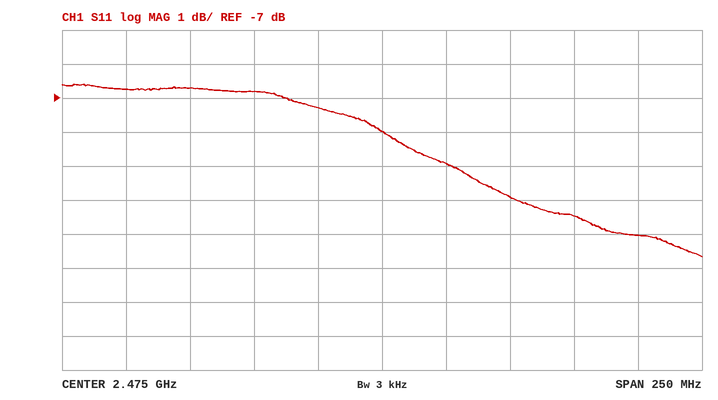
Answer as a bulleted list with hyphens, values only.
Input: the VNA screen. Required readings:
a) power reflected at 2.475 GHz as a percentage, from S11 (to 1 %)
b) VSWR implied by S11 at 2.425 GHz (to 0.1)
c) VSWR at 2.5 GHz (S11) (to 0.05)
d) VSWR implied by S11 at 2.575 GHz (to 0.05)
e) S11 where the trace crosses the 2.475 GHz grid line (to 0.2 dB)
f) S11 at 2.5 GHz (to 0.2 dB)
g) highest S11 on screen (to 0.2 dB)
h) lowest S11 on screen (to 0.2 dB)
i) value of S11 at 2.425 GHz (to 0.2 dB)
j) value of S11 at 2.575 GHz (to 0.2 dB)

- 16 %
- 2.7
- 2.10
- 1.80
- -8.0 dB
- -9.0 dB
- -6.6 dB
- -11.6 dB
- -6.8 dB
- -11.0 dB
